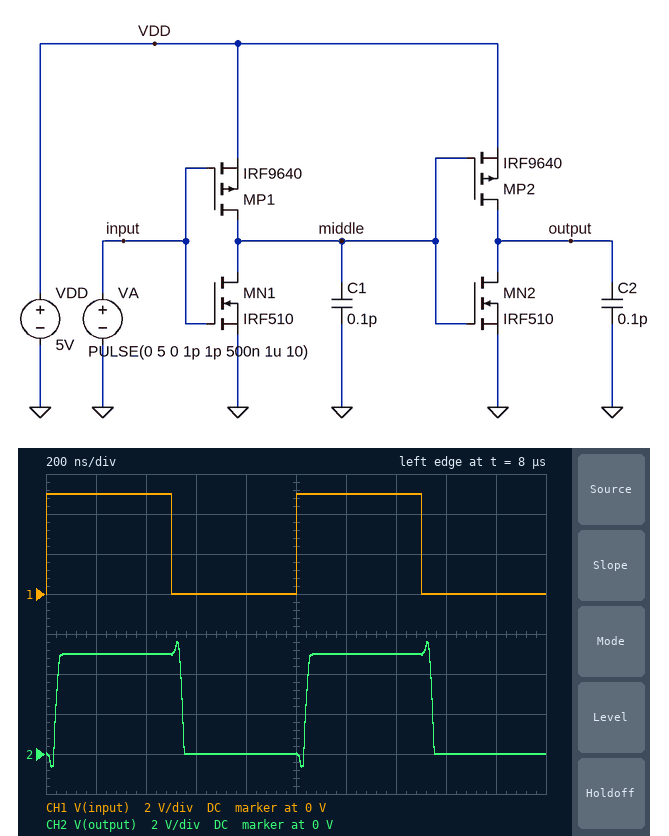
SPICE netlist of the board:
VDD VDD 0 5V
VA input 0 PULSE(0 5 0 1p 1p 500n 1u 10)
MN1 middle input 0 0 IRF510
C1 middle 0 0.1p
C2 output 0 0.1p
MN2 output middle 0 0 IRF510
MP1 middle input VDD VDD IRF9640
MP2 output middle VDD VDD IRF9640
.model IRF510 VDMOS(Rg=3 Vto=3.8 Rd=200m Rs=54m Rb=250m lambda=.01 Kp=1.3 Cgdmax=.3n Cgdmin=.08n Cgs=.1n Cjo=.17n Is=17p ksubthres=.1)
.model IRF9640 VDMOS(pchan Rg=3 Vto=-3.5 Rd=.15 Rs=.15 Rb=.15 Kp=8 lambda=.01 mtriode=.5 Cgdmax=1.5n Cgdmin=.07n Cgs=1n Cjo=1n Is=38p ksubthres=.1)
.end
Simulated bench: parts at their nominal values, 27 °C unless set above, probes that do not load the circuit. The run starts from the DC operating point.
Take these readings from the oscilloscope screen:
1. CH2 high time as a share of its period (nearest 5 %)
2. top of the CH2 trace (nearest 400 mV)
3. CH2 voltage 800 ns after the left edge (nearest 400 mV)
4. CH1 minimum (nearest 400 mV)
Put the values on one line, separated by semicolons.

50 %; 5.6 V; 0 V; 0 V
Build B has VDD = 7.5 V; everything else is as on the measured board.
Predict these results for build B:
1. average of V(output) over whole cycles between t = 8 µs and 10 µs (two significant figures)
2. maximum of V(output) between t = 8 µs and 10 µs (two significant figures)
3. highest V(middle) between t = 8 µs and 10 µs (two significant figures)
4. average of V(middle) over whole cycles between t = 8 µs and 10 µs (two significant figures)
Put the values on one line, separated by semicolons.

3.6 V; 7.7 V; 7.8 V; 3.9 V
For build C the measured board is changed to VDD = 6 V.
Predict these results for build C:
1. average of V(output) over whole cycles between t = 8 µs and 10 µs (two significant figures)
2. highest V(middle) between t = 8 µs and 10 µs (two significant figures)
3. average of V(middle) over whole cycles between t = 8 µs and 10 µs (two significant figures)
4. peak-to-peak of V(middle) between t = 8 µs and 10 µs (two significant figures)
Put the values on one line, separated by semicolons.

2.9 V; 6.3 V; 3.1 V; 7.0 V
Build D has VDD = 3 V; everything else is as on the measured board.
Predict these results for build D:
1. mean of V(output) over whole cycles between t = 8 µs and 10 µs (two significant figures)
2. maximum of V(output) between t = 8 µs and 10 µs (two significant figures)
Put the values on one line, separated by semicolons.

3.1 V; 3.3 V
